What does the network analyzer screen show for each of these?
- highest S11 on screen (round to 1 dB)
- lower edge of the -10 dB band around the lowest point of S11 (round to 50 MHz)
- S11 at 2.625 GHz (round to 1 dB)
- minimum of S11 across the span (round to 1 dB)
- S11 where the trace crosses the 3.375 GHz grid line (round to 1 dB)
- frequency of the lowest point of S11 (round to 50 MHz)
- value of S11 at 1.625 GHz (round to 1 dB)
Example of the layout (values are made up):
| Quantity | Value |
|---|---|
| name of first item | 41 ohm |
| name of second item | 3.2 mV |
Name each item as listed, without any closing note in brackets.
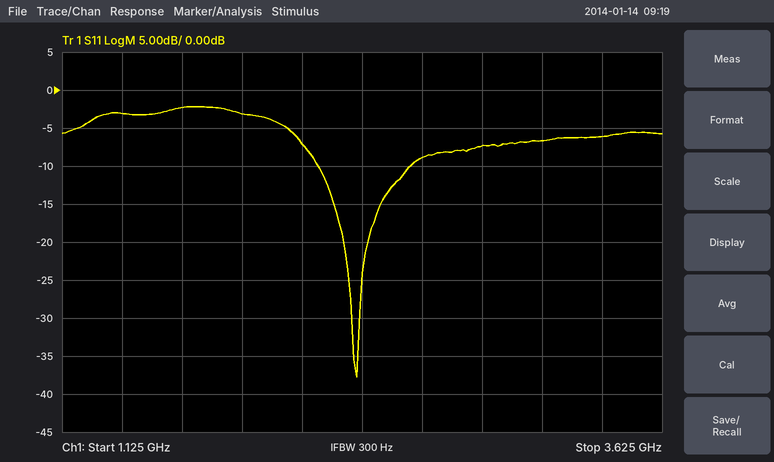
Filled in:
| Quantity | Value |
|---|---|
| highest S11 on screen | -2 dB |
| lower edge of the -10 dB band around the lowest point of S11 | 2.20 GHz |
| S11 at 2.625 GHz | -9 dB |
| minimum of S11 across the span | -38 dB |
| S11 where the trace crosses the 3.375 GHz grid line | -6 dB |
| frequency of the lowest point of S11 | 2.35 GHz |
| value of S11 at 1.625 GHz | -2 dB |
